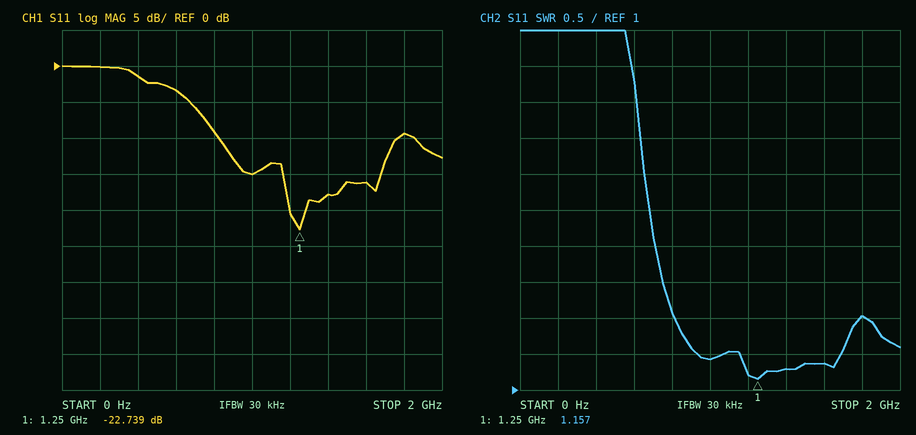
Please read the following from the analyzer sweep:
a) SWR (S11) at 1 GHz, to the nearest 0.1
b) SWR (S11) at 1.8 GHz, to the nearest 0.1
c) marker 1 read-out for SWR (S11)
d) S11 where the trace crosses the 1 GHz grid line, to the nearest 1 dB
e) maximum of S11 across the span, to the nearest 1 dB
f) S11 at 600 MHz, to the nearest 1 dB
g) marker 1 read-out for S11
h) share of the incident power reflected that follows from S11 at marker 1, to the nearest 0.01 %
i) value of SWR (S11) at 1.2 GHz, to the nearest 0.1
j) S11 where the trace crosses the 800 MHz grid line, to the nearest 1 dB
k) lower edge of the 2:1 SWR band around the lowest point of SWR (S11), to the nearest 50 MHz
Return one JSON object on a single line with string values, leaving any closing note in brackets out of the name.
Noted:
{"SWR (S11) at 1 GHz, to the nearest 0.1": "1.4", "SWR (S11) at 1.8 GHz, to the nearest 0.1": "2.0", "marker 1 read-out for SWR": "1.157", "S11 where the trace crosses the 1 GHz grid line, to the nearest 1 dB": "-15 dB", "maximum of S11 across the span, to the nearest 1 dB": "0 dB", "S11 at 600 MHz, to the nearest 1 dB": "-3 dB", "marker 1 read-out for S11": "-22.739 dB", "share of the incident power reflected that follows from S11 at marker 1, to the nearest 0.01 %": "0.53 %", "value of SWR (S11) at 1.2 GHz, to the nearest 0.1": "1.2", "S11 where the trace crosses the 800 MHz grid line, to the nearest 1 dB": "-9 dB", "lower edge of the 2:1 SWR band around the lowest point of SWR (S11), to the nearest 50 MHz": "800 MHz"}
